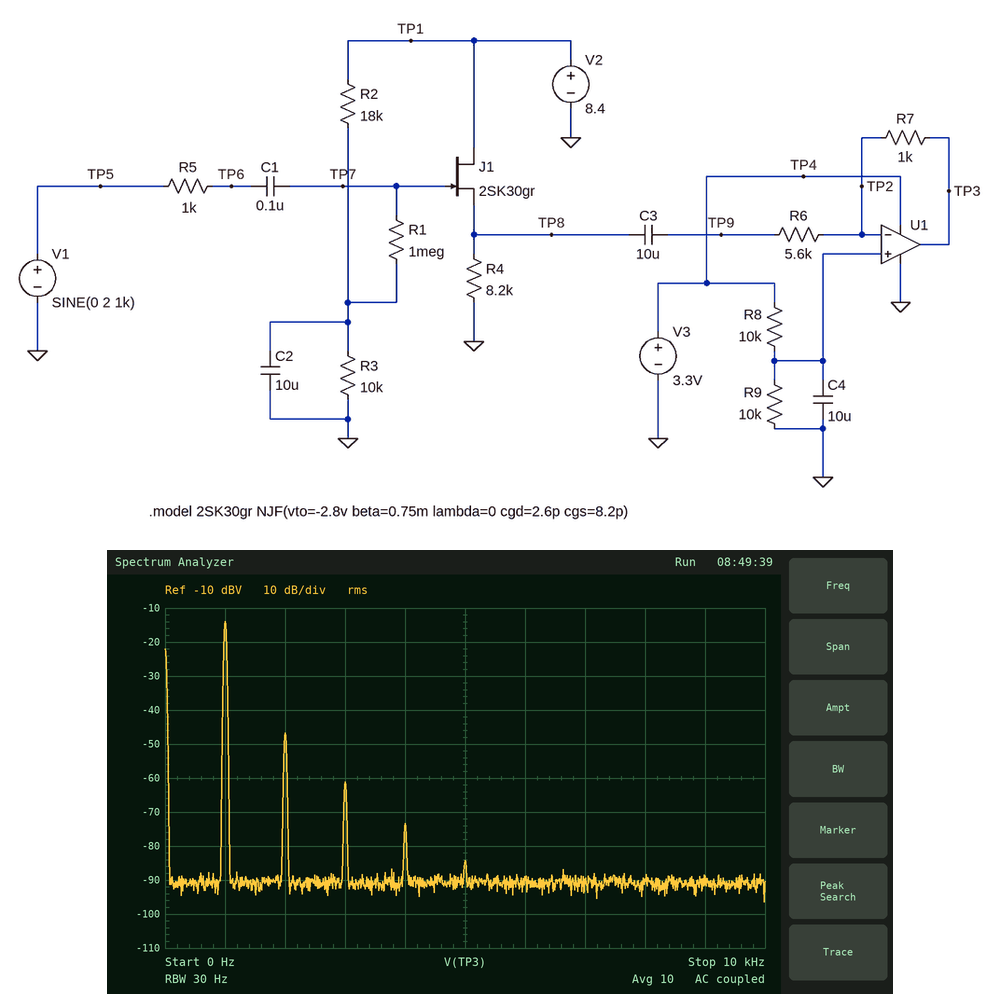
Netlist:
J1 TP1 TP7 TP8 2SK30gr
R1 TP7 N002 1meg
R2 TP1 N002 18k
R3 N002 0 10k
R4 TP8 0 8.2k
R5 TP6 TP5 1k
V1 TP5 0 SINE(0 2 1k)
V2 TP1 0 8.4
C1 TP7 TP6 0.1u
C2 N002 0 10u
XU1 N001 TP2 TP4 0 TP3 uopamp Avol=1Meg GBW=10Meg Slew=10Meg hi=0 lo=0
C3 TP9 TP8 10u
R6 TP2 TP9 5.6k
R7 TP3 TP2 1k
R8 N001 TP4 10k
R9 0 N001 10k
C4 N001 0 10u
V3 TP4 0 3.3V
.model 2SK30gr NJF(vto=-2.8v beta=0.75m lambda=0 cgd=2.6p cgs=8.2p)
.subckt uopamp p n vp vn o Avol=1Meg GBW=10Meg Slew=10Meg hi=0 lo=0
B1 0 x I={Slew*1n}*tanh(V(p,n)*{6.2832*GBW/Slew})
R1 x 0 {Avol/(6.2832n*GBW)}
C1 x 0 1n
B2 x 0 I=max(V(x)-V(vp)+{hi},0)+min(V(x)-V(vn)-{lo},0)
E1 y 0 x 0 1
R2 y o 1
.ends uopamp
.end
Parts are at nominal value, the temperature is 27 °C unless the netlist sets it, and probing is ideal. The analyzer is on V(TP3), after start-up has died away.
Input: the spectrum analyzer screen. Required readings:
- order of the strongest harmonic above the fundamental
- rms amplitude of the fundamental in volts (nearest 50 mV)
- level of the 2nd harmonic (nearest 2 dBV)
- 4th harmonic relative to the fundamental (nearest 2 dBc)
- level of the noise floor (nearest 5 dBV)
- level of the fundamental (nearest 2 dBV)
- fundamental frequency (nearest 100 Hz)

2
200 mV
-46 dBV
-60 dBc
-90 dBV
-14 dBV
1.0 kHz
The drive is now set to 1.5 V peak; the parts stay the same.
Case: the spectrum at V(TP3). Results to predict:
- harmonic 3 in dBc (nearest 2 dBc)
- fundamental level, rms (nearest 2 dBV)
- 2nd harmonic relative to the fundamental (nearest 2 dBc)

-54 dBc
-16 dBV
-36 dBc
